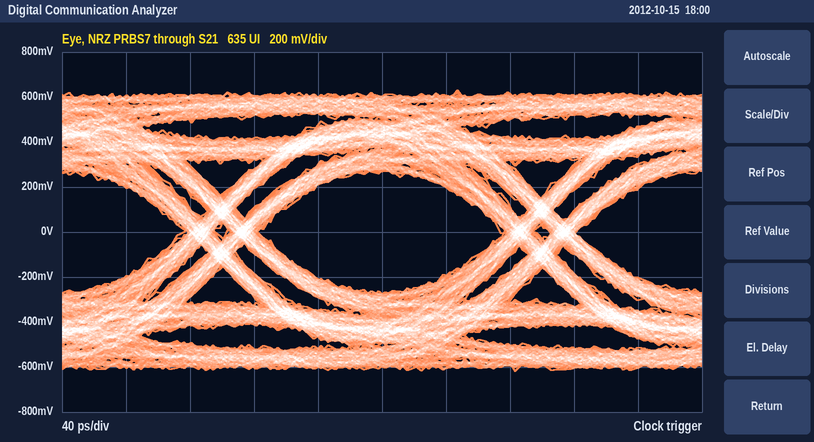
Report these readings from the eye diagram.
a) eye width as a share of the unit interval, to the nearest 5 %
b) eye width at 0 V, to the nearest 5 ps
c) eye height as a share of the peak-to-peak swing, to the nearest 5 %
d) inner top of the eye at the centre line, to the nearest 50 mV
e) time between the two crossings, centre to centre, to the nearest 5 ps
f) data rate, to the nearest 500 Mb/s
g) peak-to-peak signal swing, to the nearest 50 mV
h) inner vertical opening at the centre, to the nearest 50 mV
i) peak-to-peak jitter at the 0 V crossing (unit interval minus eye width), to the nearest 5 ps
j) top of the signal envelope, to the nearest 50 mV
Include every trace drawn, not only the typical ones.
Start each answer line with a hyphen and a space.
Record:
- 75 %
- 150 ps
- 45 %
- 250 mV
- 200 ps
- 5.0 Gb/s
- 1.25 V
- 550 mV
- 50 ps
- 650 mV
